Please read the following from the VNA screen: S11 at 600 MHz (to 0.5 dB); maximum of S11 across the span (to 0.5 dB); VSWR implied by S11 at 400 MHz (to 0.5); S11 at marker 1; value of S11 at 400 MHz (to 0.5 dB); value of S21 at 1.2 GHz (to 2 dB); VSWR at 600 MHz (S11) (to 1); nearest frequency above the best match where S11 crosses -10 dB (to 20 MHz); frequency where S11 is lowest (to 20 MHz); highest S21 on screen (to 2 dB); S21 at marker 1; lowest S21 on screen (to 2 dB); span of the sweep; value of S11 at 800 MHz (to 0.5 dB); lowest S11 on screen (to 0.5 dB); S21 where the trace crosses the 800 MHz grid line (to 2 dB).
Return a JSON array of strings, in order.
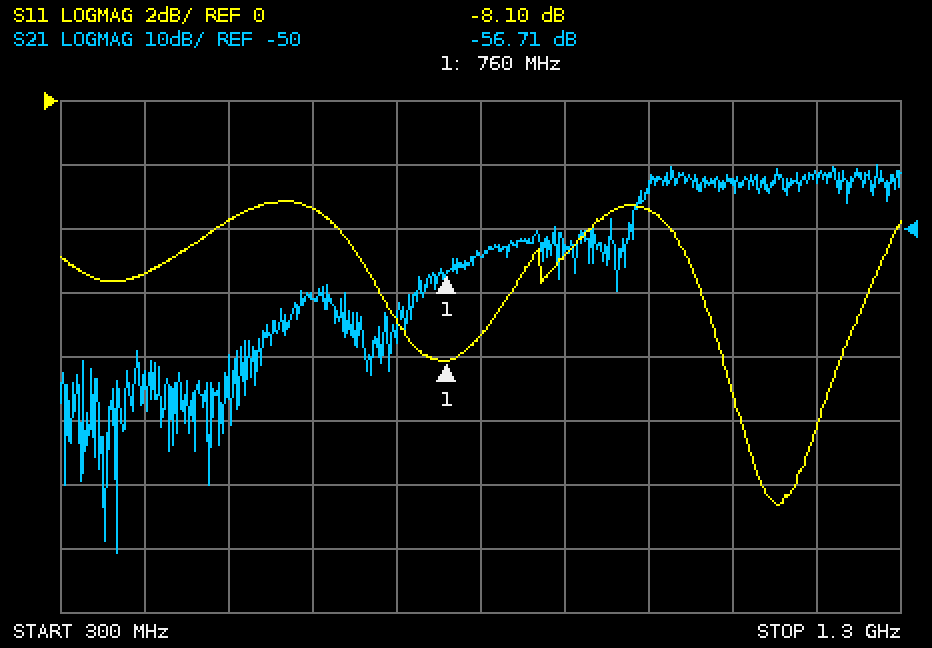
["-3.5 dB", "-3.0 dB", "3.5", "-8.10 dB", "-5.5 dB", "-42 dB", "5", "1.20 GHz", "1.16 GHz", "-40 dB", "-56.71 dB", "-100 dB", "1 GHz", "-7.5 dB", "-12.5 dB", "-54 dB"]
